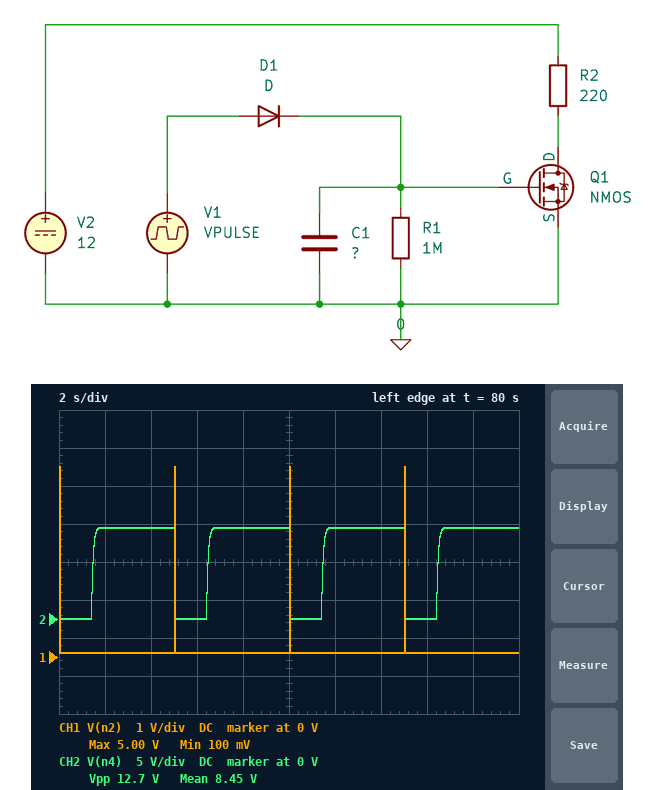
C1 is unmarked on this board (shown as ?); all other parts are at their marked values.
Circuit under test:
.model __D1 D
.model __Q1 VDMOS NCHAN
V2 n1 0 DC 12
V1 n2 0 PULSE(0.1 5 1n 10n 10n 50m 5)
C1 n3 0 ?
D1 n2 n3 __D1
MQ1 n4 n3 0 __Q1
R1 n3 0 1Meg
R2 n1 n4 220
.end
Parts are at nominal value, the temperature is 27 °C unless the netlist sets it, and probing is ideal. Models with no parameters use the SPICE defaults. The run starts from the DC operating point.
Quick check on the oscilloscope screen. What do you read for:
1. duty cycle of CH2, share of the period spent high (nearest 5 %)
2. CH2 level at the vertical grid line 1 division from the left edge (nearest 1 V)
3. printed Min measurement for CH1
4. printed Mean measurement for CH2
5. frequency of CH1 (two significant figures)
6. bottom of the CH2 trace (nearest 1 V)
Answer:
70 %
12 V
100 mV
8.45 V
200 mHz
0 V
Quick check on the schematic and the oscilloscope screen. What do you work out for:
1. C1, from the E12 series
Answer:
3.3 µF
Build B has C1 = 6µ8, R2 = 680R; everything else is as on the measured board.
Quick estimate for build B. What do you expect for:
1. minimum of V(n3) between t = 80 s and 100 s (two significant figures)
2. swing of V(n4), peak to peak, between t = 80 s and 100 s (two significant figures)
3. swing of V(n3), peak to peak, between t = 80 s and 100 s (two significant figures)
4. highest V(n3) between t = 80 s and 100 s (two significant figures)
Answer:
2.2 V
12 V
2.3 V
4.5 V
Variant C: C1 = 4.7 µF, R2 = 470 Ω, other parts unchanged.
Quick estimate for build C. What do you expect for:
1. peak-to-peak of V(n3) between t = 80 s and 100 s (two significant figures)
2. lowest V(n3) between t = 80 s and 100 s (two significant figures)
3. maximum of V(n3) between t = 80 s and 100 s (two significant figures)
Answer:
2.9 V
1.6 V
4.5 V
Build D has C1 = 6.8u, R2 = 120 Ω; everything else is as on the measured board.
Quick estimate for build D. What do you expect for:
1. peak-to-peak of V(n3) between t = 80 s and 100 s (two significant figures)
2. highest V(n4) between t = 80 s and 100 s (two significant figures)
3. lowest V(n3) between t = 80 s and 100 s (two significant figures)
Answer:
2.3 V
12 V
2.2 V
